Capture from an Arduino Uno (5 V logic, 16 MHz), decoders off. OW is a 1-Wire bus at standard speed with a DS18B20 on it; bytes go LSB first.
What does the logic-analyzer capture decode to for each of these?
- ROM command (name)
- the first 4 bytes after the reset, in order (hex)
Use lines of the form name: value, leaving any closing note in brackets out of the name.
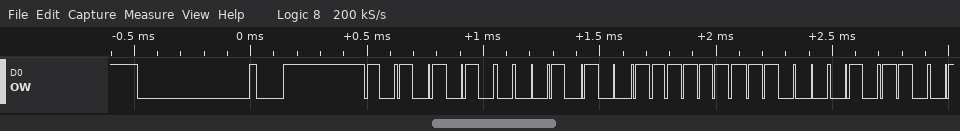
ROM command: Match ROM
the first 4 bytes after the reset, in order: 55 28 FF A1
